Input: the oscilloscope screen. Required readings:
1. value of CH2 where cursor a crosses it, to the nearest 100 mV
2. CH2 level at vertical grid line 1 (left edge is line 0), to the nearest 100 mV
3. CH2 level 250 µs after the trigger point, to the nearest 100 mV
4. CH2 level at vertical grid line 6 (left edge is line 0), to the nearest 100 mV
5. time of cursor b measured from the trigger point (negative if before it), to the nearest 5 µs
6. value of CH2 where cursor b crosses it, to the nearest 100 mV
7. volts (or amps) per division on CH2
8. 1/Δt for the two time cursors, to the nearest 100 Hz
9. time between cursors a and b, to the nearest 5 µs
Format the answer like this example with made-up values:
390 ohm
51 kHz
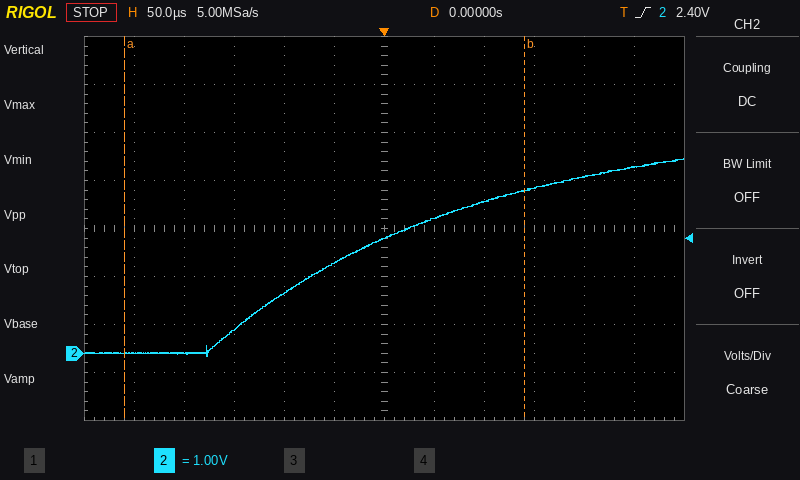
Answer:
0.0 V
0.0 V
3.9 V
2.4 V
+140 µs
3.4 V
1 V
2.5 kHz
400 µs
